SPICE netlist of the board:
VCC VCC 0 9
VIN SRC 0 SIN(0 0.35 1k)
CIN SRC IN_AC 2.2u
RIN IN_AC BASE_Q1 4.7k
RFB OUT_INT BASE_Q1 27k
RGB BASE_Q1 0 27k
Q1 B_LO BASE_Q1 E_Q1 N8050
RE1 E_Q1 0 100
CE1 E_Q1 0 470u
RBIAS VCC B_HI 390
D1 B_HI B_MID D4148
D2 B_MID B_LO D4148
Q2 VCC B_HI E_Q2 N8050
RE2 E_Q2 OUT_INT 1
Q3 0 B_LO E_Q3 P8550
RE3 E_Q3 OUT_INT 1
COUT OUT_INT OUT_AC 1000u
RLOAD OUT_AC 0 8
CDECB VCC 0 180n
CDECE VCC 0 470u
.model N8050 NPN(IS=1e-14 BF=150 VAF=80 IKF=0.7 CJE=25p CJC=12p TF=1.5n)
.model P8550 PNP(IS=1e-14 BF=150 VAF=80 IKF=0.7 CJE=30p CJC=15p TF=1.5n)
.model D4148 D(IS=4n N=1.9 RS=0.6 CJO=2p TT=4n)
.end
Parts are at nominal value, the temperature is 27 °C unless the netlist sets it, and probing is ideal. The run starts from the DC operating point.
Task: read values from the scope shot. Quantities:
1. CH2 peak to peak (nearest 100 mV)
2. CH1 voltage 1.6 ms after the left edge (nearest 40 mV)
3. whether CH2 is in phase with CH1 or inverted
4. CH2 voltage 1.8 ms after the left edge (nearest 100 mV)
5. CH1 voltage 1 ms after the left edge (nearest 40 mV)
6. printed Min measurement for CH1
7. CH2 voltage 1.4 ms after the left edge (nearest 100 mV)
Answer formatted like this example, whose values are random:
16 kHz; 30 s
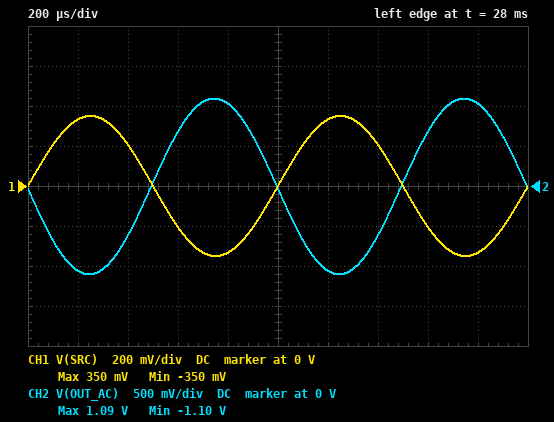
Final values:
2.2 V; -200 mV; inverted; 1.0 V; 0 V; -350 mV; -600 mV
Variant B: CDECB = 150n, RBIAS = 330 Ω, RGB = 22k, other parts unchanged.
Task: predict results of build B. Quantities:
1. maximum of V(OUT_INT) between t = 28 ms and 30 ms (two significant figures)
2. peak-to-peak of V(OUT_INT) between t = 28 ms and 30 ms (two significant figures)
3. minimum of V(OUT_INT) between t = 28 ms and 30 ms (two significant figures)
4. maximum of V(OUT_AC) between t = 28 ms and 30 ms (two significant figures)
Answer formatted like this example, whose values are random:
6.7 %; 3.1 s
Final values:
6.3 V; 2.1 V; 4.2 V; 1.0 V
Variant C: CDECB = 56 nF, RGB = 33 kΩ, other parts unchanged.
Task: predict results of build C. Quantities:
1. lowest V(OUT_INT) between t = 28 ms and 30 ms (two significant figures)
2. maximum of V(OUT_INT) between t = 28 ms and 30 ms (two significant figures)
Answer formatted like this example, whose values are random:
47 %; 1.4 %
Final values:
3.5 V; 5.7 V
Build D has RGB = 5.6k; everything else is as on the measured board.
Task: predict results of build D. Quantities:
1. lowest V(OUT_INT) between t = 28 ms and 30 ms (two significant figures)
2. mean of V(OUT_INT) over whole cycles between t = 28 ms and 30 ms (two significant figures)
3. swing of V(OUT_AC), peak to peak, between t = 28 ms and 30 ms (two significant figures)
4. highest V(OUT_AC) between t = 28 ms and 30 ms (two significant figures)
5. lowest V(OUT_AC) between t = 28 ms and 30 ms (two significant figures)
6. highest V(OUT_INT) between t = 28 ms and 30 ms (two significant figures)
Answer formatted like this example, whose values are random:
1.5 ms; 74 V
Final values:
5.8 V; 6.8 V; 1.8 V; 840 mV; -980 mV; 7.7 V
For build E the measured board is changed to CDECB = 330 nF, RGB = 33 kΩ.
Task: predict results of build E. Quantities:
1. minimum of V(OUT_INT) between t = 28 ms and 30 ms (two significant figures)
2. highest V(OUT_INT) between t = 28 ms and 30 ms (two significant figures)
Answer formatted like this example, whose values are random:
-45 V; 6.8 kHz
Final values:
3.5 V; 5.7 V
